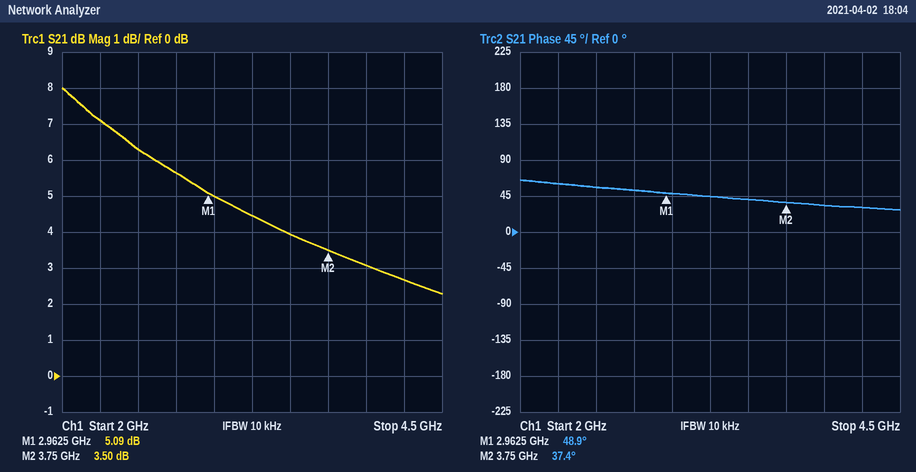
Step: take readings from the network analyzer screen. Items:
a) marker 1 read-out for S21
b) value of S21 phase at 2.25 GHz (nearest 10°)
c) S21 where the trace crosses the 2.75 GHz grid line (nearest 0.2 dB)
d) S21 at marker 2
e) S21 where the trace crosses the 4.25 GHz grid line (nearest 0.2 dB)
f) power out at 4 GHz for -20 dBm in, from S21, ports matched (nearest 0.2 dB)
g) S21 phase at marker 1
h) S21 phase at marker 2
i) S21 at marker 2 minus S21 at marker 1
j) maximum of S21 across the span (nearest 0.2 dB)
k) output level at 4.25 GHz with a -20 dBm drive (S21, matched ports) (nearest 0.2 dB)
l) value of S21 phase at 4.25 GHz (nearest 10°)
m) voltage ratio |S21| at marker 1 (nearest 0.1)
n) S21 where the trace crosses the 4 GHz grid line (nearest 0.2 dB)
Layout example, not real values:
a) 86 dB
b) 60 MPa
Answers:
a) 5.09 dB
b) 60°
c) 5.6 dB
d) 3.50 dB
e) 2.6 dB
f) -17.0 dBm
g) 48.9°
h) 37.4°
i) -1.59 dB
j) 8.0 dB
k) -17.4 dBm
l) 30°
m) 1.8
n) 3.0 dB
